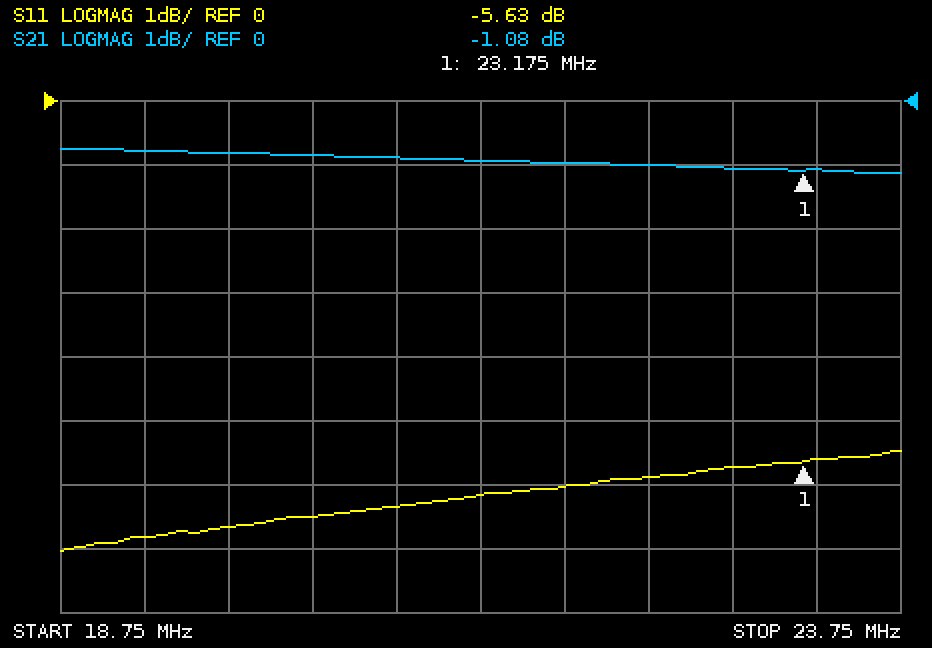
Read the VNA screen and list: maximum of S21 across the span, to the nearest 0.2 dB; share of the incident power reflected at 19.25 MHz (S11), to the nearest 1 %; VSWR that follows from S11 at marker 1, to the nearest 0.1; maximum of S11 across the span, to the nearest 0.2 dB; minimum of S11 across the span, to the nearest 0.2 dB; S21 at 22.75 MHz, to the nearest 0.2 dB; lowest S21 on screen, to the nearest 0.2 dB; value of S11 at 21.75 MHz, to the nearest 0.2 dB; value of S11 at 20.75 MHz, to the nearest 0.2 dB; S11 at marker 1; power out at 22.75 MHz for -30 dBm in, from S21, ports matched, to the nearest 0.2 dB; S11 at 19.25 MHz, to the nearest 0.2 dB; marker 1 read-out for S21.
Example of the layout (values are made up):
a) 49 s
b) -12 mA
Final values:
a) -0.8 dB
b) 21 %
c) 3.2
d) -5.4 dB
e) -7.0 dB
f) -1.0 dB
g) -1.2 dB
h) -6.0 dB
i) -6.4 dB
j) -5.63 dB
k) -31.0 dBm
l) -6.8 dB
m) -1.08 dB
